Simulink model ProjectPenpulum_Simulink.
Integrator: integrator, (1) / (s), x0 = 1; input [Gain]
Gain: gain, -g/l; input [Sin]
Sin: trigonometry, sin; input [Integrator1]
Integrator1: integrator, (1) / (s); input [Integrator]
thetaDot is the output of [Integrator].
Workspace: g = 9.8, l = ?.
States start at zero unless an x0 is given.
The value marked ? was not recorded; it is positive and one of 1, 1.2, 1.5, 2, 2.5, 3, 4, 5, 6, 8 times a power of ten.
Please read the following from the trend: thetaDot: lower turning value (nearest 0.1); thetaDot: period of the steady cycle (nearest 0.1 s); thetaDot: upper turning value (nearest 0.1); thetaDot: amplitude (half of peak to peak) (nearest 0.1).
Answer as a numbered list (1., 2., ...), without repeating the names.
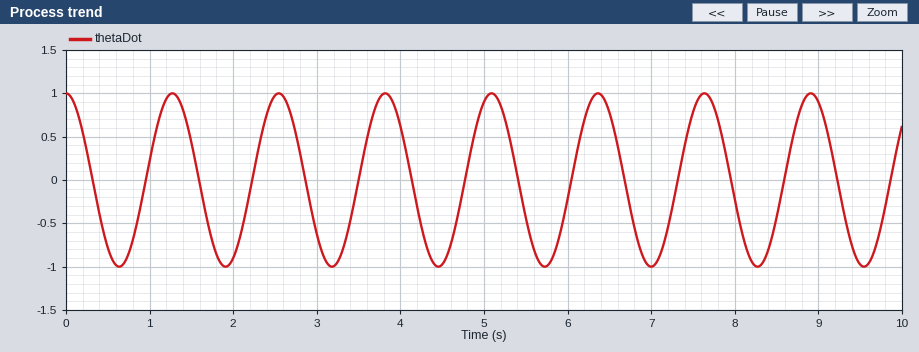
1. -1.0
2. 1.3 s
3. 1.0
4. 1.0
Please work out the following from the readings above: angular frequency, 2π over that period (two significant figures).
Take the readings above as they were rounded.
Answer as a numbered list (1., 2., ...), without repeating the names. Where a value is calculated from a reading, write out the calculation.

1. 2π / 1.3 = 4.8 rad/s
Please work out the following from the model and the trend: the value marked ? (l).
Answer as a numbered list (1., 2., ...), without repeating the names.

1. 0.4
